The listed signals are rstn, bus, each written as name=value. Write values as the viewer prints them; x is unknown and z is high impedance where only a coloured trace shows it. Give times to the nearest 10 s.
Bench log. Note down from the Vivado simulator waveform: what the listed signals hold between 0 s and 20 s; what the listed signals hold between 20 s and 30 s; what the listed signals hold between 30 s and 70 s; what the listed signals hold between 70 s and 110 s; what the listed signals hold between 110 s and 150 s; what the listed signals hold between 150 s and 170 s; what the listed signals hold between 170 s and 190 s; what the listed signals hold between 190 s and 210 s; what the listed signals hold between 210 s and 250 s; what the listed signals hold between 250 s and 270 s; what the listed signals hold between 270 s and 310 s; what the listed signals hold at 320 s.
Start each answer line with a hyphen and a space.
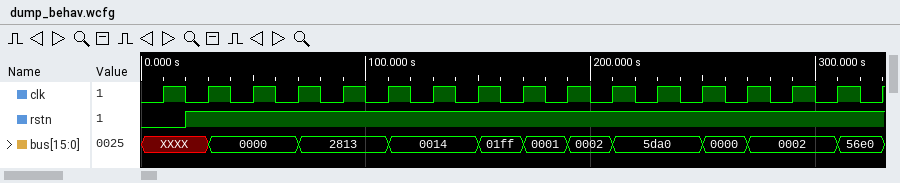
- rstn=0, bus=XXXX
- rstn=1, bus=XXXX
- rstn=1, bus=0000
- rstn=1, bus=2813
- rstn=1, bus=0014
- rstn=1, bus=01ff
- rstn=1, bus=0001
- rstn=1, bus=0002
- rstn=1, bus=5da0
- rstn=1, bus=0000
- rstn=1, bus=0002
- rstn=1, bus=56e0
